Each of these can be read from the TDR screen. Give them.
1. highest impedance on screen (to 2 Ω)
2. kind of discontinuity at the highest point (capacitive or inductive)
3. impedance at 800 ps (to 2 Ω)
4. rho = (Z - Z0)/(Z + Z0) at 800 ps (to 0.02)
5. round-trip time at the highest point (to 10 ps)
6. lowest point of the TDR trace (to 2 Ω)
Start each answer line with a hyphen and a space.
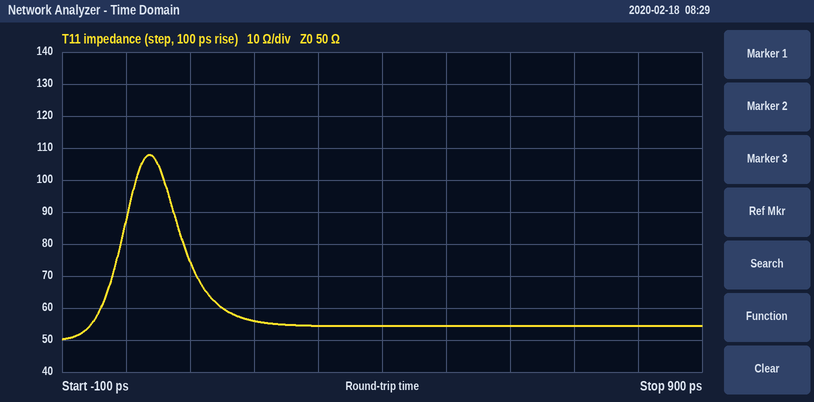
- 108 Ω
- inductive
- 54 Ω
- +0.04
- 40 ps
- 50 Ω
